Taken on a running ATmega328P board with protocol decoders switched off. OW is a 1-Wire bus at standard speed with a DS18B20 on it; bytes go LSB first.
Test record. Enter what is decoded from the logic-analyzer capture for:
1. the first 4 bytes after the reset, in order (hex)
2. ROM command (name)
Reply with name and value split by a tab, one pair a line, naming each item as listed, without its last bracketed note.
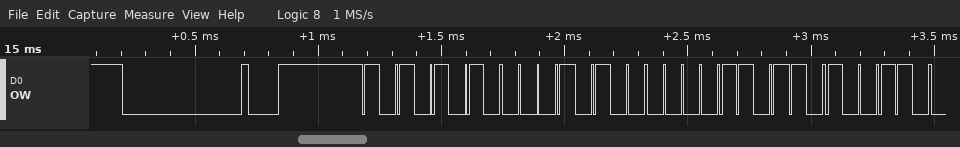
the first 4 bytes after the reset, in order	55 28 B0 65
ROM command	Match ROM
